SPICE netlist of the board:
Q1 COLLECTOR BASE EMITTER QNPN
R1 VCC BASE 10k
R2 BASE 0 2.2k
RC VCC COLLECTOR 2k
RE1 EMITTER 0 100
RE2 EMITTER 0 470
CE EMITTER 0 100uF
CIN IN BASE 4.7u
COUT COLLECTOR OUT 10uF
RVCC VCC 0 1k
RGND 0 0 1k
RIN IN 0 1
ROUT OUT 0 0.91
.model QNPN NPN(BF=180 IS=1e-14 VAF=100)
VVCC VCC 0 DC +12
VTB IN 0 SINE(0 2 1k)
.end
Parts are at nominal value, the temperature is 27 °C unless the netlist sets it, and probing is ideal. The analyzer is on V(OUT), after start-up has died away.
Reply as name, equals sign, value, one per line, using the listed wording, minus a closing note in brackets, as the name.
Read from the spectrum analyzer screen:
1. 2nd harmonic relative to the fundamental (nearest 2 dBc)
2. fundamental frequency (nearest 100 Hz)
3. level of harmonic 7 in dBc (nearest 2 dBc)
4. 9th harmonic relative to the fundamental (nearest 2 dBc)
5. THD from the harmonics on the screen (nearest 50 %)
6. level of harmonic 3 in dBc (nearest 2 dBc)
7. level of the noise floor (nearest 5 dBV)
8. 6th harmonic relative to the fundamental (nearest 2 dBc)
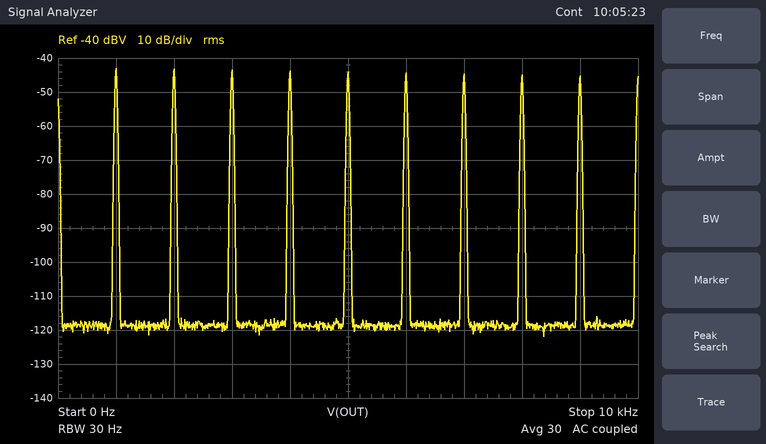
2nd harmonic relative to the fundamental = 0 dBc
fundamental frequency = 1.0 kHz
level of harmonic 7 in dBc = -2 dBc
9th harmonic relative to the fundamental = -2 dBc
THD from the harmonics on the screen = 250 %
level of harmonic 3 in dBc = 0 dBc
level of the noise floor = -120 dBV
6th harmonic relative to the fundamental = -2 dBc
